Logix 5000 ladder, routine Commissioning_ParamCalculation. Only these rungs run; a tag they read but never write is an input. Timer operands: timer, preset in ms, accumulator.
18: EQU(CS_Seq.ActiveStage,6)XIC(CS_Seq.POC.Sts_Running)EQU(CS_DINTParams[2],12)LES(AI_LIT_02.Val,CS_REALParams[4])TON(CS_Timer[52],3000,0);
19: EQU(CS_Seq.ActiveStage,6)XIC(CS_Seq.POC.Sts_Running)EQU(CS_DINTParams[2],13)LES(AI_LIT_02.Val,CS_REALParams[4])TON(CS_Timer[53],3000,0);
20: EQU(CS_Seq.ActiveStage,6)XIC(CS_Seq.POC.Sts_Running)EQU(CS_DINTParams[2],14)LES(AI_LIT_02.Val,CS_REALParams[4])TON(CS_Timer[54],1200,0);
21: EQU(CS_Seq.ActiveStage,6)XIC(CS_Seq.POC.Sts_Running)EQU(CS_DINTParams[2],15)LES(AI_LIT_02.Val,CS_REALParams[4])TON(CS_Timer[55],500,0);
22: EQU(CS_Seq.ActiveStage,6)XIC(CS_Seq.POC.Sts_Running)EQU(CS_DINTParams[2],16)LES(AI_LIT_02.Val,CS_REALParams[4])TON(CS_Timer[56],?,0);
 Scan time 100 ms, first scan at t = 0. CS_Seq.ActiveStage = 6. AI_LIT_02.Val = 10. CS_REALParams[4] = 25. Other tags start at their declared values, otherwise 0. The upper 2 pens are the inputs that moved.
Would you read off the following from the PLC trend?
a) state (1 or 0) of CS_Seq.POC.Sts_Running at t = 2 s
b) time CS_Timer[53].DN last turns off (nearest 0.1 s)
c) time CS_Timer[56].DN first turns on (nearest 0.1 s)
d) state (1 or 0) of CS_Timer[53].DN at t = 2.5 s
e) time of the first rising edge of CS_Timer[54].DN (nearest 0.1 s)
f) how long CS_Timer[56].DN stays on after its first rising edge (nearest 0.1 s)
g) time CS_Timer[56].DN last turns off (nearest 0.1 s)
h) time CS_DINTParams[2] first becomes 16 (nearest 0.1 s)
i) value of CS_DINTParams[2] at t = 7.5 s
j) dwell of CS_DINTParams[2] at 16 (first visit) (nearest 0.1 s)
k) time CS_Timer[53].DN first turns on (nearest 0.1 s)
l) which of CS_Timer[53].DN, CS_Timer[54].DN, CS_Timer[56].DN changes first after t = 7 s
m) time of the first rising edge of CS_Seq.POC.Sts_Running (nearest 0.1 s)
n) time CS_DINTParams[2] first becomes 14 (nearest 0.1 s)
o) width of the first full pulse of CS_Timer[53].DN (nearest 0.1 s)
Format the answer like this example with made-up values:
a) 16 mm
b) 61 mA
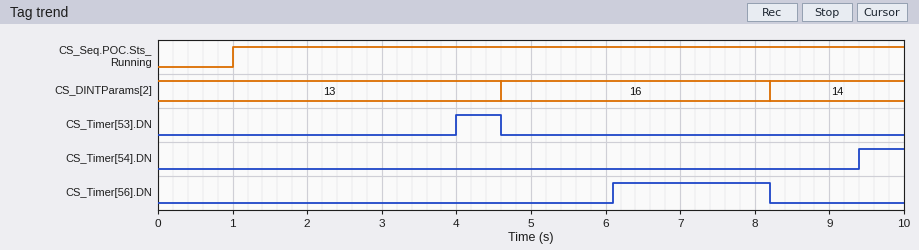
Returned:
a) 1
b) 4.6 s
c) 6.1 s
d) 0
e) 9.4 s
f) 2.1 s
g) 8.2 s
h) 4.6 s
i) 16
j) 3.6 s
k) 4.0 s
l) CS_Timer[56].DN
m) 1.0 s
n) 8.2 s
o) 0.6 s
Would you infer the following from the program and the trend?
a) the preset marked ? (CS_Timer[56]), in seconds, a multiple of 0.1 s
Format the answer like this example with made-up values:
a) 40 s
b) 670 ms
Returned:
a) 1.5 s
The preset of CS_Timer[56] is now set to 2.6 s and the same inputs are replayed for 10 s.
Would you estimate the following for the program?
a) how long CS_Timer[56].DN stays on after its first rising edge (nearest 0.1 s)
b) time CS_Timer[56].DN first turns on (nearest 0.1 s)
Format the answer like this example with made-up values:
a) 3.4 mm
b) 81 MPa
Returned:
a) 1.0 s
b) 7.2 s
